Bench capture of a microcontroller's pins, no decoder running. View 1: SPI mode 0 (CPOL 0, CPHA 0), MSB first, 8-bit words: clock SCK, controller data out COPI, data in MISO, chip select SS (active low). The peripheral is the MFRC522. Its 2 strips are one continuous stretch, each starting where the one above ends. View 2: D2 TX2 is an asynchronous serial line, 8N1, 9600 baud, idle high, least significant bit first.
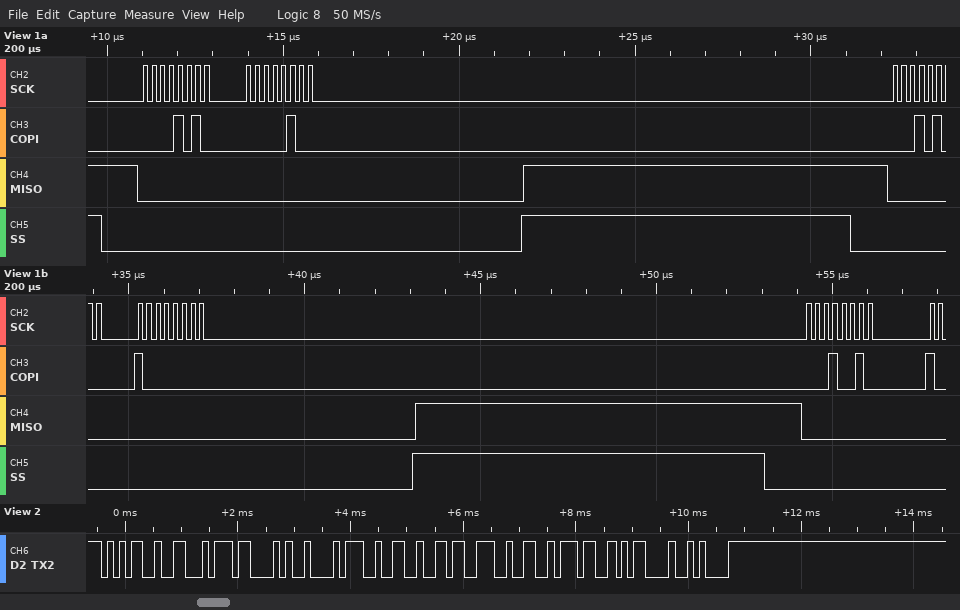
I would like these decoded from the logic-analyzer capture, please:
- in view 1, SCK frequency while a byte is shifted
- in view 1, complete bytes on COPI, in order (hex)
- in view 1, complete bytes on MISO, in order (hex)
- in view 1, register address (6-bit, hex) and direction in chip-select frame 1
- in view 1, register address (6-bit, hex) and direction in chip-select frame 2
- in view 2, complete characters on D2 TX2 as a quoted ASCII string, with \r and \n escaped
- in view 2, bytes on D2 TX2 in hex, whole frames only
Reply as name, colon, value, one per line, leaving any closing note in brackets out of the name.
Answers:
in view 1, SCK frequency while a byte is shifted: 4 MHz
in view 1, complete bytes on COPI, in order: 0A 04 14 80 12
in view 1, complete bytes on MISO, in order: 00 00 00 00 00
in view 1, register address (6-bit, hex) and direction in chip-select frame 1: 0x05 write
in view 1, register address (6-bit, hex) and direction in chip-select frame 2: 0x0A write
in view 2, complete characters on D2 TX2 as a quoted ASCII string, with \r and \n escaped: "5FCB2627\r\n"
in view 2, bytes on D2 TX2 in hex, whole frames only: 0x35 0x46 0x43 0x42 0x32 0x36 0x32 0x37 0x0D 0x0A
